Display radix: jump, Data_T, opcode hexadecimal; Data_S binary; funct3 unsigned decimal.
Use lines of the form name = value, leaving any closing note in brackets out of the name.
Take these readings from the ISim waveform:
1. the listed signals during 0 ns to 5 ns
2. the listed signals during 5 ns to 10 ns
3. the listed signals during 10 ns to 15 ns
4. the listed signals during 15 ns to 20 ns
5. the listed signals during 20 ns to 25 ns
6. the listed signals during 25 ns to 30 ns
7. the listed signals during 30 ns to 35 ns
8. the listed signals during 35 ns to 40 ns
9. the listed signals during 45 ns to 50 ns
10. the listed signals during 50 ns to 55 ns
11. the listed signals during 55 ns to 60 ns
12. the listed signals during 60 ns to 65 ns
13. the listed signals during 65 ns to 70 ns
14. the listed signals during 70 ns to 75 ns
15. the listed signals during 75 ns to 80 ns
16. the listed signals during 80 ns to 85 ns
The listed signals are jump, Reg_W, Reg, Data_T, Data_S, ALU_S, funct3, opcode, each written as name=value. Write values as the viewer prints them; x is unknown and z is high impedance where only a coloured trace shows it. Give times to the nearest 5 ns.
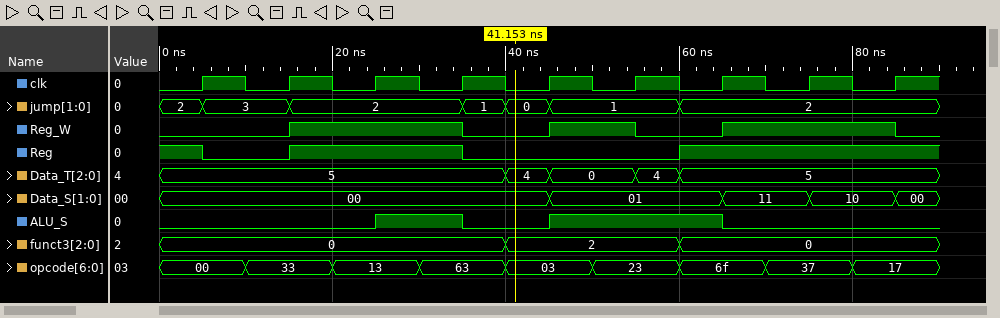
the listed signals during 0 ns to 5 ns = jump=2, Reg_W=0, Reg=1, Data_T=5, Data_S=00, ALU_S=0, funct3=0, opcode=00
the listed signals during 5 ns to 10 ns = jump=3, Reg_W=0, Reg=0, Data_T=5, Data_S=00, ALU_S=0, funct3=0, opcode=00
the listed signals during 10 ns to 15 ns = jump=3, Reg_W=0, Reg=0, Data_T=5, Data_S=00, ALU_S=0, funct3=0, opcode=33
the listed signals during 15 ns to 20 ns = jump=2, Reg_W=1, Reg=1, Data_T=5, Data_S=00, ALU_S=0, funct3=0, opcode=33
the listed signals during 20 ns to 25 ns = jump=2, Reg_W=1, Reg=1, Data_T=5, Data_S=00, ALU_S=0, funct3=0, opcode=13
the listed signals during 25 ns to 30 ns = jump=2, Reg_W=1, Reg=1, Data_T=5, Data_S=00, ALU_S=1, funct3=0, opcode=13
the listed signals during 30 ns to 35 ns = jump=2, Reg_W=1, Reg=1, Data_T=5, Data_S=00, ALU_S=1, funct3=0, opcode=63
the listed signals during 35 ns to 40 ns = jump=1, Reg_W=0, Reg=0, Data_T=5, Data_S=00, ALU_S=0, funct3=0, opcode=63
the listed signals during 45 ns to 50 ns = jump=1, Reg_W=1, Reg=0, Data_T=0, Data_S=01, ALU_S=1, funct3=2, opcode=03
the listed signals during 50 ns to 55 ns = jump=1, Reg_W=1, Reg=0, Data_T=0, Data_S=01, ALU_S=1, funct3=2, opcode=23
the listed signals during 55 ns to 60 ns = jump=1, Reg_W=0, Reg=0, Data_T=4, Data_S=01, ALU_S=1, funct3=2, opcode=23
the listed signals during 60 ns to 65 ns = jump=2, Reg_W=0, Reg=1, Data_T=5, Data_S=01, ALU_S=1, funct3=0, opcode=6f
the listed signals during 65 ns to 70 ns = jump=2, Reg_W=1, Reg=1, Data_T=5, Data_S=11, ALU_S=0, funct3=0, opcode=6f
the listed signals during 70 ns to 75 ns = jump=2, Reg_W=1, Reg=1, Data_T=5, Data_S=11, ALU_S=0, funct3=0, opcode=37
the listed signals during 75 ns to 80 ns = jump=2, Reg_W=1, Reg=1, Data_T=5, Data_S=10, ALU_S=0, funct3=0, opcode=37
the listed signals during 80 ns to 85 ns = jump=2, Reg_W=1, Reg=1, Data_T=5, Data_S=10, ALU_S=0, funct3=0, opcode=17
